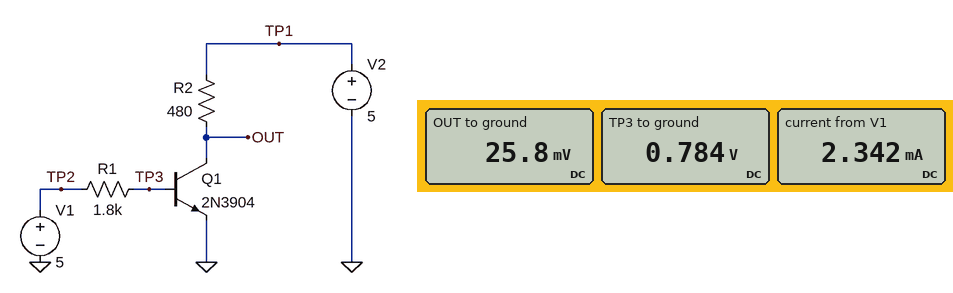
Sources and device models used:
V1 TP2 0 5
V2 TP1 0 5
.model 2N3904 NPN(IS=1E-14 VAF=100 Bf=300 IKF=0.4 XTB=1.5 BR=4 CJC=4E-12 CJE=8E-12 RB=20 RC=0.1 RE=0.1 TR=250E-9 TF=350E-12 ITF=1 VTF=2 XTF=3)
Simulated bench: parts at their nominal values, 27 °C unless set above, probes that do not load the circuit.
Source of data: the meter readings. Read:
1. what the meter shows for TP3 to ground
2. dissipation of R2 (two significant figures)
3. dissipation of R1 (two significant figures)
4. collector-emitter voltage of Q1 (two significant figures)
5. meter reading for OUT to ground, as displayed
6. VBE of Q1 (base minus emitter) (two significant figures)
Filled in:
0.784 V
52 mW
9.9 mW
26 mV
25.8 mV
780 mV
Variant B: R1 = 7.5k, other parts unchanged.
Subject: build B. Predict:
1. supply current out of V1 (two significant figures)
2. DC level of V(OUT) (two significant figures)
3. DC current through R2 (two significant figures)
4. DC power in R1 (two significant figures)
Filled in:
570 µA
50 mV
10 mA
2.4 mW
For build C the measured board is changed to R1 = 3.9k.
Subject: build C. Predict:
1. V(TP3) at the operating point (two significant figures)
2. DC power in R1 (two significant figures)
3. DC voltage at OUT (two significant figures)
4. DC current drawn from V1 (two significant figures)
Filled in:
750 mV
4.6 mW
37 mV
1.1 mA
